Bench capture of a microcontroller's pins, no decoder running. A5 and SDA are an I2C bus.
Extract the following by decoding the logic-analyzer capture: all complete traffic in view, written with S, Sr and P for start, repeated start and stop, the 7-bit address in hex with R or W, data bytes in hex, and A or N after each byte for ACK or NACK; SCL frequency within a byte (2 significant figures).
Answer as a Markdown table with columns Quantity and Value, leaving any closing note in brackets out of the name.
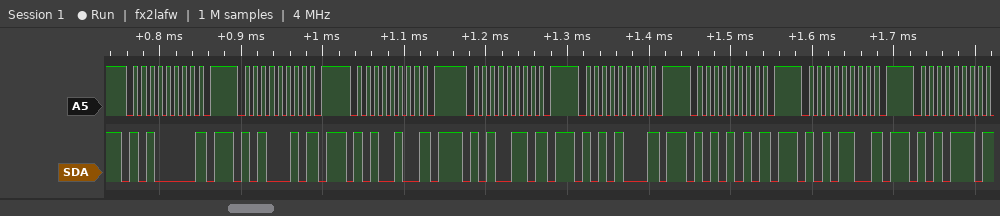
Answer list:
| Quantity | Value |
|---|---|
| all complete traffic in view, written with S, Sr and P for start, repeated start and stop, the 7-bit address in hex with R or W, data bytes in hex, and A or N after each byte for ACK or NACK | S 50W N P S 51W N P S 52W N P S 53W N P S 54W N P S 55W N P S 56W N P S 57W N |
| SCL frequency within a byte | 100 kHz |
